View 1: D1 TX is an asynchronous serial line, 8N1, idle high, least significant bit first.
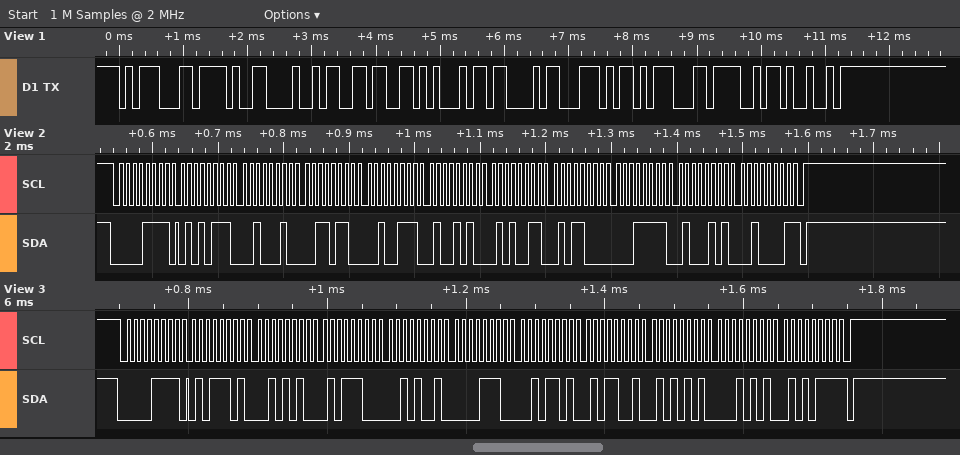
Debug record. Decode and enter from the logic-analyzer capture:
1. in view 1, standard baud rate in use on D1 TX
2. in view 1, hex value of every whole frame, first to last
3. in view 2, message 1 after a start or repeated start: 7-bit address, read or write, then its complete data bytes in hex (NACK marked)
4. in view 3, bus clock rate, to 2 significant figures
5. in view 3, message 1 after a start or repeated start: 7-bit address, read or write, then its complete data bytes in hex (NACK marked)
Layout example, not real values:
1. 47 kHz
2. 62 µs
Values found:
1. 9600 baud
2. 1D 2F 48 36 45 43 5C 1D 4F 49
3. 0x07 read: 57 22 36 27 4A 53 58 1F 45 21 NACK
4. 100 kHz
5. 0x07 read: 5D 2A 5C 29 0E 2D 59 55 15 57 NACK
